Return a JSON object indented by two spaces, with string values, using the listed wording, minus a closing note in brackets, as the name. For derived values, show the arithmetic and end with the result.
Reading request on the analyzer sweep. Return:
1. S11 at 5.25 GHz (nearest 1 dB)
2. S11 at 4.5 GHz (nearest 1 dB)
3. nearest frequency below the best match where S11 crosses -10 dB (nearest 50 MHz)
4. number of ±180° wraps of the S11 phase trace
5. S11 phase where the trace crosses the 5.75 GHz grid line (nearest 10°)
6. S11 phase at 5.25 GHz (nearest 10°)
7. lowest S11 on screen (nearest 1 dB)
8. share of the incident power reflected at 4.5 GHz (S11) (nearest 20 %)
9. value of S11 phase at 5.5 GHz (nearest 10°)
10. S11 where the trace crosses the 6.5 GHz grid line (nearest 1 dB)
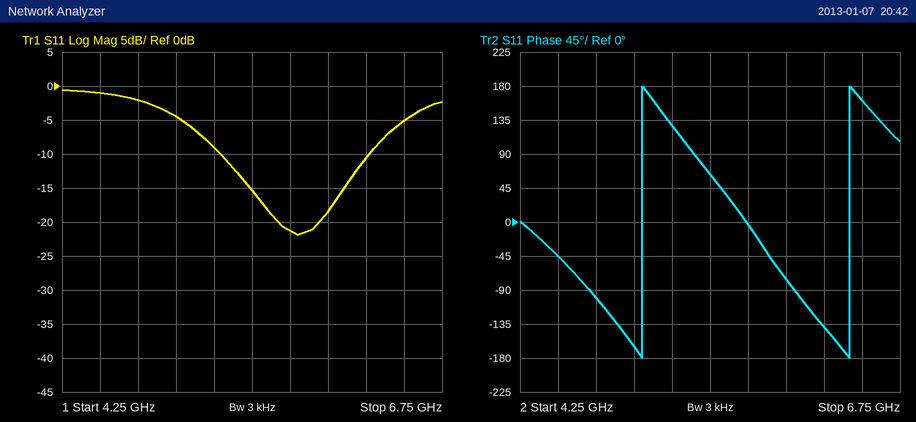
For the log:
{
  "S11 at 5.25 GHz": "-9 dB",
  "S11 at 4.5 GHz": "-1 dB",
  "nearest frequency below the best match where S11 crosses -10 dB": "5.30 GHz",
  "number of ±180° wraps of the S11 phase trace": "2",
  "S11 phase where the trace crosses the 5.75 GHz grid line": "0°",
  "S11 phase at 5.25 GHz": "130°",
  "lowest S11 on screen": "-22 dB",
  "share of the incident power reflected at 4.5 GHz (S11)": "10^(-1/10) ≈ 79.4 %, so 80 % to the nearest 20 %",
  "value of S11 phase at 5.5 GHz": "60°",
  "S11 where the trace crosses the 6.5 GHz grid line": "-5 dB"
}
